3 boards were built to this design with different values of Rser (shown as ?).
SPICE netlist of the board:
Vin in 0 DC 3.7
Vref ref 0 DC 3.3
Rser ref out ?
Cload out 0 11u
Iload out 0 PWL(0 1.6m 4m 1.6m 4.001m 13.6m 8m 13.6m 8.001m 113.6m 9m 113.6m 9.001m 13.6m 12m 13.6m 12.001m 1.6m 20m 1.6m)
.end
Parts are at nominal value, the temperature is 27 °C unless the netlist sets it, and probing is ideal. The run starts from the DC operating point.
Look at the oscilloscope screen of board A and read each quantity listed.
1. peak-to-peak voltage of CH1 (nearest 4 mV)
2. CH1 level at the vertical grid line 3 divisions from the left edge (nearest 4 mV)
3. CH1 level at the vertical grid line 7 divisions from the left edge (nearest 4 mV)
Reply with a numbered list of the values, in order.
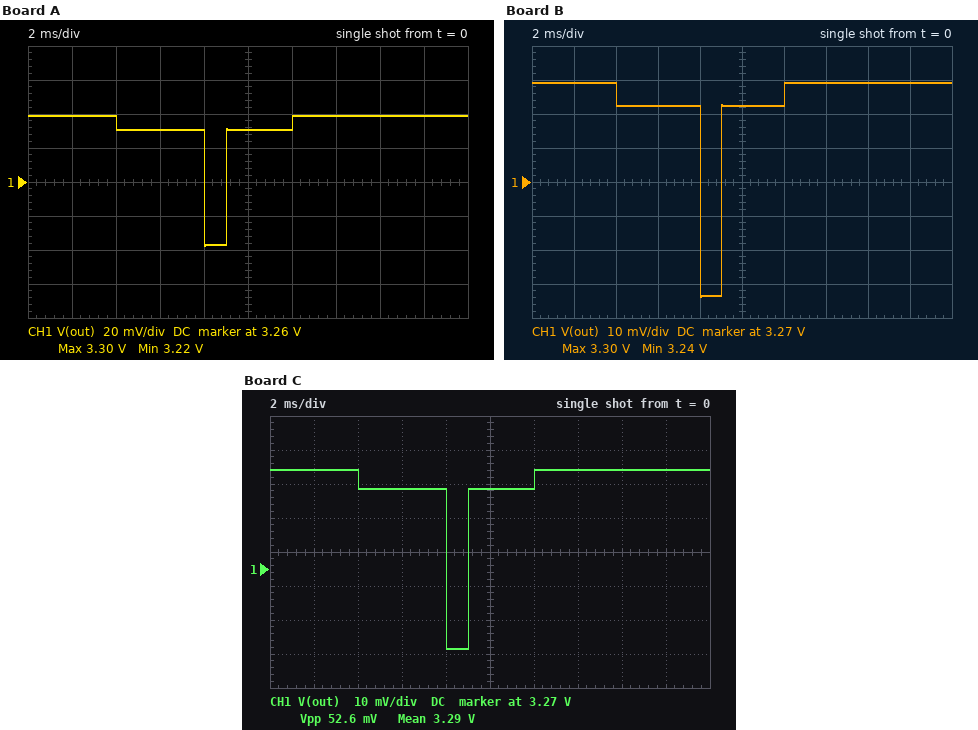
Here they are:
1. 76 mV
2. 3.292 V
3. 3.300 V
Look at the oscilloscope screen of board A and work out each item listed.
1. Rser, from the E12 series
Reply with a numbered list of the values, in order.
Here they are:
1. 0.68 Ω
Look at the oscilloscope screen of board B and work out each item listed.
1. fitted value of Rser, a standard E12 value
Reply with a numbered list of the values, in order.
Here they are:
1. 0.56 Ω
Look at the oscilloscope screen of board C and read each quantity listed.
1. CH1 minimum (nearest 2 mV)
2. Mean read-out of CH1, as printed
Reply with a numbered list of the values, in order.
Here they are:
1. 3.246 V
2. 3.29 V
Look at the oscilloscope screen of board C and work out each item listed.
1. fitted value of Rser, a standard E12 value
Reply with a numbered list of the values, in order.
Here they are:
1. 0.47 Ω
